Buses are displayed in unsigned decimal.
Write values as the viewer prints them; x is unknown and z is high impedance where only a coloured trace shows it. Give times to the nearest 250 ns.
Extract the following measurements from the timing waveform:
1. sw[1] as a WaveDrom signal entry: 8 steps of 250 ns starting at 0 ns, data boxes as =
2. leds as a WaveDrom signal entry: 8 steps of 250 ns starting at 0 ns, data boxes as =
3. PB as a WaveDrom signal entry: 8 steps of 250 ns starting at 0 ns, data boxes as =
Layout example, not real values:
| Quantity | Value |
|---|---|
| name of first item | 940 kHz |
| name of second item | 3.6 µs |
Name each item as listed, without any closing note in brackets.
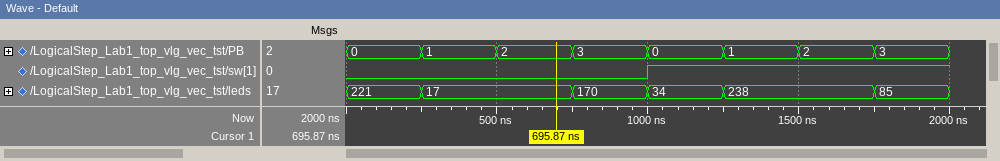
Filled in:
| Quantity | Value |
|---|---|
| sw[1] as a WaveDrom signal entry: 8 steps of 250 ns starting at 0 ns, data boxes as = | {name: 'sw[1]', wave: '0...1...'} |
| leds as a WaveDrom signal entry: 8 steps of 250 ns starting at 0 ns, data boxes as = | {name: 'leds', wave: '==.===.=', data: '221 17 170 34 238 85'} |
| PB as a WaveDrom signal entry: 8 steps of 250 ns starting at 0 ns, data boxes as = | {name: 'PB', wave: '========', data: '0 1 2 3 0 1 2 3'} |
